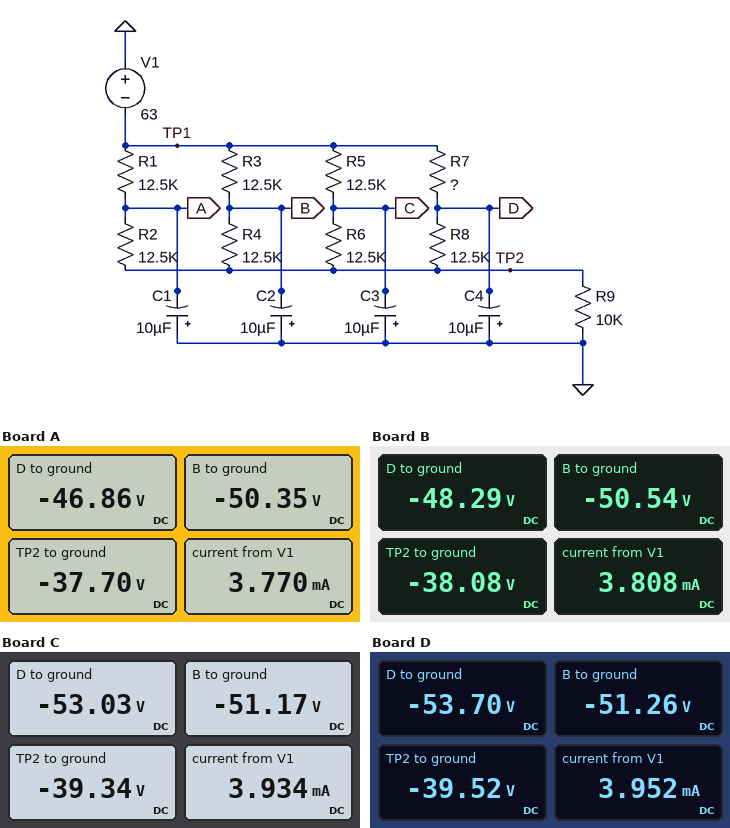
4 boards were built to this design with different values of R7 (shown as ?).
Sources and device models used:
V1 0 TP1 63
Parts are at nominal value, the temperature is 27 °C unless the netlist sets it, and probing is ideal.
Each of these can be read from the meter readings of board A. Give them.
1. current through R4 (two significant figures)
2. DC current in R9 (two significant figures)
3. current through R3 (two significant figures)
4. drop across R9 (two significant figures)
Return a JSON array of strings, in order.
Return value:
["1.0 mA", "3.8 mA", "1.0 mA", "38 V"]
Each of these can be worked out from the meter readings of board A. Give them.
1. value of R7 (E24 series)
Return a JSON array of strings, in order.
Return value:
["22 kΩ"]
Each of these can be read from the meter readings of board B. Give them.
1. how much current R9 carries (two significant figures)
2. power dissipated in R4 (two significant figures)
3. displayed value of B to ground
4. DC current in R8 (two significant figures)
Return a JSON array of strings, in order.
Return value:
["3.8 mA", "12 mW", "-50.54 V", "820 µA"]
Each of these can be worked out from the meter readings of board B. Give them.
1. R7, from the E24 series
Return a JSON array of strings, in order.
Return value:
["18 kΩ"]
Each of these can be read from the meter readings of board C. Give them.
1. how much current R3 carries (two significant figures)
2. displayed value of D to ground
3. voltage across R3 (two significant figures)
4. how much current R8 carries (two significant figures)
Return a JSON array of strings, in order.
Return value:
["950 µA", "-53.03 V", "12 V", "1.1 mA"]
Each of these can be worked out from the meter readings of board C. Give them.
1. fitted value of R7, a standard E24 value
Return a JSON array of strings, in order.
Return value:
["9.1 kΩ"]
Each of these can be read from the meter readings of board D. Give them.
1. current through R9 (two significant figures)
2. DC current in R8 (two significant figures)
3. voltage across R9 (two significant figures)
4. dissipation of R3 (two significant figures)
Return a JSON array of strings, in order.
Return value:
["4.0 mA", "1.1 mA", "40 V", "11 mW"]
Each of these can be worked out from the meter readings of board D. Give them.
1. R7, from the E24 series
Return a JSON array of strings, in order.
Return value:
["8.2 kΩ"]
